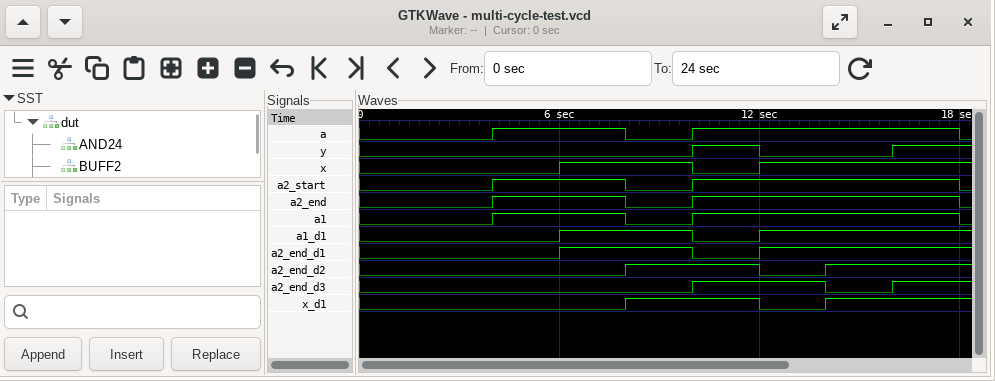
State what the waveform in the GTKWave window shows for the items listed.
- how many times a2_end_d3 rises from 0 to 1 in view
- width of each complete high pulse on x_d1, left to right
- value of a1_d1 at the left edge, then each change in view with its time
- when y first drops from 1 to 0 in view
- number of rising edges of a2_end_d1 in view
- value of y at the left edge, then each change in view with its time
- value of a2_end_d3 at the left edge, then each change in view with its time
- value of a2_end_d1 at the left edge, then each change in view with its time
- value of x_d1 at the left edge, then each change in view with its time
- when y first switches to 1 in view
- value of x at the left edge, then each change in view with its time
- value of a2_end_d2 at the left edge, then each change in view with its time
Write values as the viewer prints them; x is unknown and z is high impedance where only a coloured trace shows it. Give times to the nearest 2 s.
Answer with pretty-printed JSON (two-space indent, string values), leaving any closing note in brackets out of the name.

{
  "how many times a2_end_d3 rises from 0 to 1 in view": "2",
  "width of each complete high pulse on x_d1, left to right": "4 s",
  "value of a1_d1 at the left edge, then each change in view with its time": "0, 1 at 6 s, 0 at 10 s, 1 at 12 s",
  "when y first drops from 1 to 0 in view": "12 s",
  "number of rising edges of a2_end_d1 in view": "2",
  "value of y at the left edge, then each change in view with its time": "0, 1 at 10 s, 0 at 12 s, 1 at 16 s",
  "value of a2_end_d3 at the left edge, then each change in view with its time": "0, 1 at 10 s, 0 at 14 s, 1 at 16 s",
  "value of a2_end_d1 at the left edge, then each change in view with its time": "0, 1 at 6 s, 0 at 10 s, 1 at 12 s",
  "value of x_d1 at the left edge, then each change in view with its time": "0, 1 at 8 s, 0 at 12 s, 1 at 14 s",
  "when y first switches to 1 in view": "10 s",
  "value of x at the left edge, then each change in view with its time": "0, 1 at 6 s, 0 at 10 s, 1 at 12 s",
  "value of a2_end_d2 at the left edge, then each change in view with its time": "0, 1 at 8 s, 0 at 12 s, 1 at 14 s"
}
